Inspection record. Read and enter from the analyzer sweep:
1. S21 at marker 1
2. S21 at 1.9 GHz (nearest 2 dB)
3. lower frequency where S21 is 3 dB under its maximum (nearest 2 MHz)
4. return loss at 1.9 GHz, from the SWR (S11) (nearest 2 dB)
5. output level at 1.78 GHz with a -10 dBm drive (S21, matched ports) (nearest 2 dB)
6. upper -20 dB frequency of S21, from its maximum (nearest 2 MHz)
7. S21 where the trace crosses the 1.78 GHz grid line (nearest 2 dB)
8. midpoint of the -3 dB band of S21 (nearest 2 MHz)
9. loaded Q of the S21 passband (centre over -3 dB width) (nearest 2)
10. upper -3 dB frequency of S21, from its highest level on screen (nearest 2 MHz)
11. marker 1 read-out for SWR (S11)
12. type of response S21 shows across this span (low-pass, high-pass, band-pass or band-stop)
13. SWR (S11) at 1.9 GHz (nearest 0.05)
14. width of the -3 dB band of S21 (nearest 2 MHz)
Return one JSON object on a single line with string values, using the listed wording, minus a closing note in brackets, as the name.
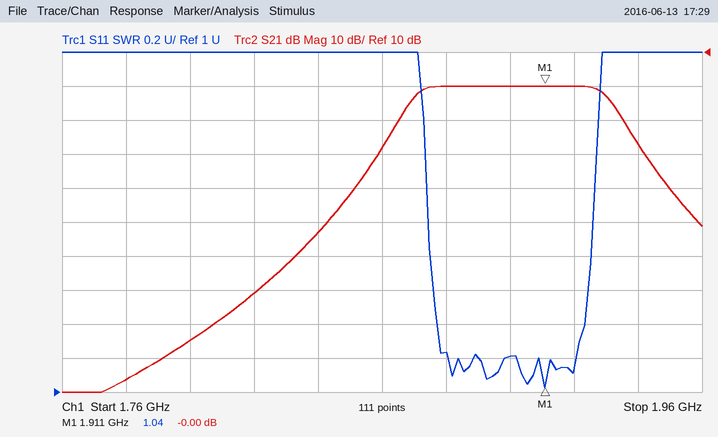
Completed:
{"S21 at marker 1": "-0.00 dB", "S21 at 1.9 GHz": "0 dB", "lower frequency where S21 is 3 dB under its maximum": "1.870 GHz", "return loss at 1.9 GHz, from the SWR (S11)": "20 dB", "output level at 1.78 GHz with a -10 dBm drive (S21, matched ports)": "-96 dBm", "upper -20 dB frequency of S21, from its maximum": "1.942 GHz", "S21 where the trace crosses the 1.78 GHz grid line": "-86 dB", "midpoint of the -3 dB band of S21": "1.900 GHz", "loaded Q of the S21 passband (centre over -3 dB width)": "32", "upper -3 dB frequency of S21, from its highest level on screen": "1.930 GHz", "marker 1 read-out for SWR": "1.04", "type of response S21 shows across this span": "band-pass", "SWR (S11) at 1.9 GHz": "1.20", "width of the -3 dB band of S21": "60 MHz"}
